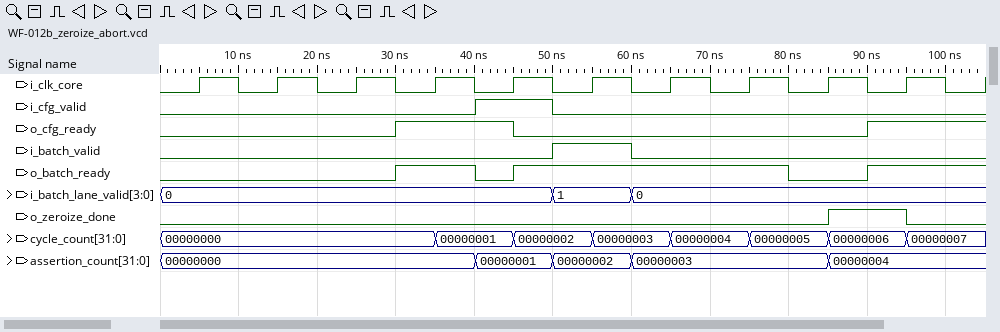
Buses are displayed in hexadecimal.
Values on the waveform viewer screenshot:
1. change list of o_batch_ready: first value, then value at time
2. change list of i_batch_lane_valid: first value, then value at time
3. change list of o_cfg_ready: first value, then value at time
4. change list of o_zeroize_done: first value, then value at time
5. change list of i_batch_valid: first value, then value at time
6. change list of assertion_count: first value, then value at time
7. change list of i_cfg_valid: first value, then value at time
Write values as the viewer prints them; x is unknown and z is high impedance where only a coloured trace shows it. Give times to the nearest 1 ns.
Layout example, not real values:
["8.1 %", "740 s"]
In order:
["0, 1 at 30 ns, 0 at 40 ns, 1 at 45 ns, 0 at 80 ns, 1 at 90 ns", "0, 1 at 50 ns, 0 at 60 ns", "0, 1 at 30 ns, 0 at 45 ns, 1 at 90 ns", "0, 1 at 85 ns, 0 at 95 ns", "0, 1 at 50 ns, 0 at 60 ns", "00000000, 00000001 at 40 ns, 00000002 at 50 ns, 00000003 at 60 ns, 00000004 at 85 ns", "0, 1 at 40 ns, 0 at 50 ns"]
